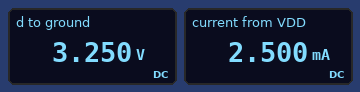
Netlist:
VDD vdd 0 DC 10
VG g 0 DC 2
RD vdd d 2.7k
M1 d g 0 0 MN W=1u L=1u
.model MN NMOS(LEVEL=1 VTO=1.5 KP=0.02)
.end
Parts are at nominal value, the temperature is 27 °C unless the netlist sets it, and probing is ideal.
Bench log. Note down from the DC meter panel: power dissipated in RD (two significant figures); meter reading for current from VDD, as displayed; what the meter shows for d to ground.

17 mW
2.500 mA
3.250 V
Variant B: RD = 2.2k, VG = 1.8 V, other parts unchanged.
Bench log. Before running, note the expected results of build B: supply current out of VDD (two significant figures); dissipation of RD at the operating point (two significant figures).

900 µA
1.8 mW
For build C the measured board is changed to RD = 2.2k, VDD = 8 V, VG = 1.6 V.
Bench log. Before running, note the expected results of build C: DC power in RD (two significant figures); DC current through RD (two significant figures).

22 µW
100 µA
